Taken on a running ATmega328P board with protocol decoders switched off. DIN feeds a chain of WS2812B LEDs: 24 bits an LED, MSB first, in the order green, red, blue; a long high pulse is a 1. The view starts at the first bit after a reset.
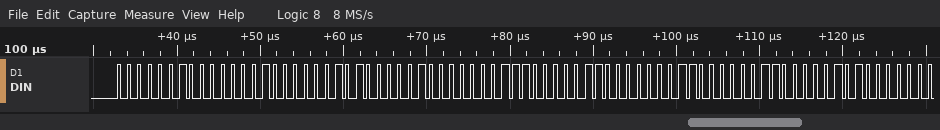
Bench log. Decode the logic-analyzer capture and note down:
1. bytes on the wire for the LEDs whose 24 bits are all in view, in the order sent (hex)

02 02 05 04 07 06 03 03 05
